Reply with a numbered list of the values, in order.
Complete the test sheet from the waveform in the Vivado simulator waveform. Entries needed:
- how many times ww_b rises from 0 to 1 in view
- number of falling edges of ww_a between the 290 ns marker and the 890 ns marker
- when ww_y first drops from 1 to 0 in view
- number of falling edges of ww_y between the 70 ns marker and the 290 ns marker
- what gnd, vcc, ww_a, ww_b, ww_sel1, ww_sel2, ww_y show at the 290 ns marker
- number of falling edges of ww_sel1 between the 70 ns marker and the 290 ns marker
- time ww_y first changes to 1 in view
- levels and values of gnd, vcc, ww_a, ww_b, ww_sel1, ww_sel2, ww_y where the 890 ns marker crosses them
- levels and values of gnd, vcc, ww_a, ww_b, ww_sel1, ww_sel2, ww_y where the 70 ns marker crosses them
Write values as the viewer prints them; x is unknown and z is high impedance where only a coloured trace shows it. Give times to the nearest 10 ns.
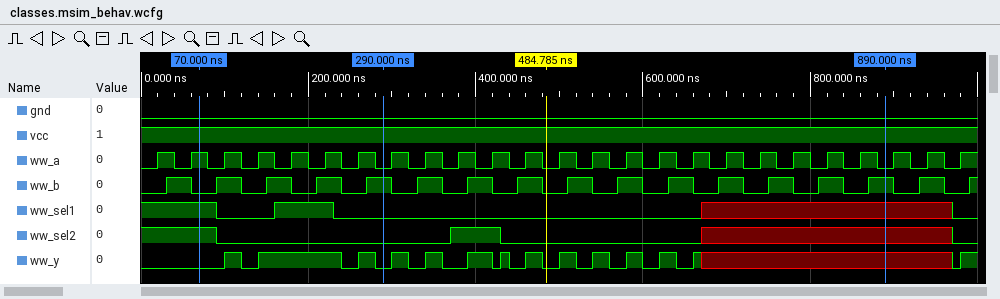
1. 17
2. 15
3. 120 ns
4. 3
5. gnd=0, vcc=1, ww_a=0, ww_b=1, ww_sel1=0, ww_sel2=0, ww_y=0
6. 2
7. 100 ns
8. gnd=0, vcc=1, ww_a=0, ww_b=1, ww_sel1=x, ww_sel2=x, ww_y=x
9. gnd=0, vcc=1, ww_a=1, ww_b=0, ww_sel1=1, ww_sel2=1, ww_y=0
